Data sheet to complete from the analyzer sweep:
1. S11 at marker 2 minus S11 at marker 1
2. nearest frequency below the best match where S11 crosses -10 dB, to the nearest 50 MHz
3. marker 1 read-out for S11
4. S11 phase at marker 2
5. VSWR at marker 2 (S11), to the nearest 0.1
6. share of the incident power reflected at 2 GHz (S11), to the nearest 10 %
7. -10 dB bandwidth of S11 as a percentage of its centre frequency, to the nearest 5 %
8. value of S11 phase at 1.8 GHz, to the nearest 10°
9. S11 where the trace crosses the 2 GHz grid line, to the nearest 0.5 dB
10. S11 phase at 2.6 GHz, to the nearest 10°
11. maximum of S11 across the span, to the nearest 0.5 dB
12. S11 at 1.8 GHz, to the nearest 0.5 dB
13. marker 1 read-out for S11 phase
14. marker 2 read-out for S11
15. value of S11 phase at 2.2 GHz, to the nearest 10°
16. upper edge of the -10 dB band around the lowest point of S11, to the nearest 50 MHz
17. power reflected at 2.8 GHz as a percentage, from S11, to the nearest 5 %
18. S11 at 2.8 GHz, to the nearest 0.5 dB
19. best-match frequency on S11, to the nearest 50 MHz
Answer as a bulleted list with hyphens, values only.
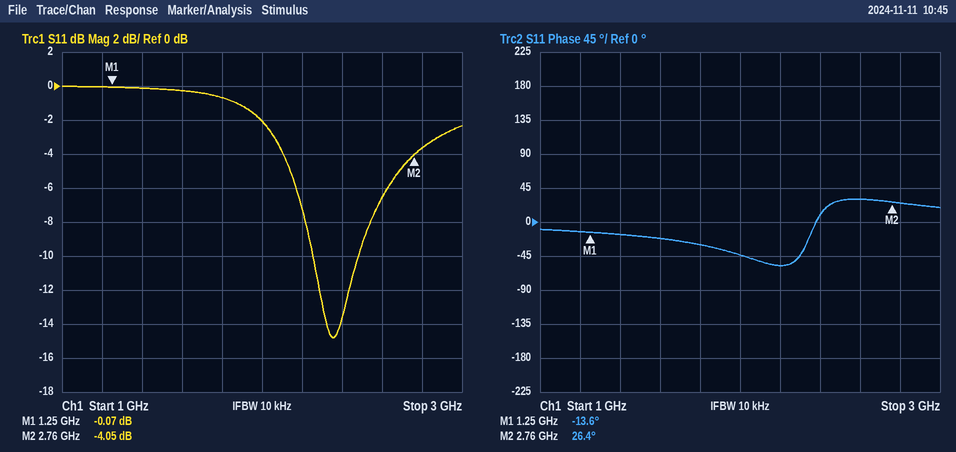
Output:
- -3.98 dB
- 2.25 GHz
- -0.07 dB
- 26.4°
- 4.4
- 60 %
- 10 %
- -30°
- -2.0 dB
- 30°
- 0.0 dB
- -0.5 dB
- -13.6°
- -4.05 dB
- -60°
- 2.50 GHz
- 45 %
- -3.5 dB
- 2.35 GHz
